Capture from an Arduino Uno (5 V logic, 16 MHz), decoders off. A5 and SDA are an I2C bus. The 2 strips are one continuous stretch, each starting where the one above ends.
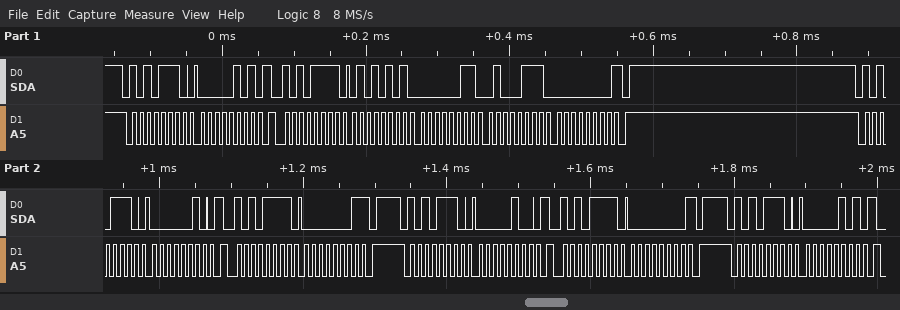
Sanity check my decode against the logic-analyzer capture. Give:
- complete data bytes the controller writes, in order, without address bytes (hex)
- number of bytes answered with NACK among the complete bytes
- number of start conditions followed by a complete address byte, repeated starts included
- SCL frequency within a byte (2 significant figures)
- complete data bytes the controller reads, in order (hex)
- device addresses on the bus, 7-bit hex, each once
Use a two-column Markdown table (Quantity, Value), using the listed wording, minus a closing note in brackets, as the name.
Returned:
| Quantity | Value |
|---|---|
| complete data bytes the controller writes, in order, without address bytes | 05 02 04 05 |
| number of bytes answered with NACK among the complete bytes | 3 |
| number of start conditions followed by a complete address byte, repeated starts included | 7 |
| SCL frequency within a byte | 100 kHz |
| complete data bytes the controller reads, in order | 55 03 47 00 01 00 |
| device addresses on the bus, 7-bit hex, each once | 0x57 |
